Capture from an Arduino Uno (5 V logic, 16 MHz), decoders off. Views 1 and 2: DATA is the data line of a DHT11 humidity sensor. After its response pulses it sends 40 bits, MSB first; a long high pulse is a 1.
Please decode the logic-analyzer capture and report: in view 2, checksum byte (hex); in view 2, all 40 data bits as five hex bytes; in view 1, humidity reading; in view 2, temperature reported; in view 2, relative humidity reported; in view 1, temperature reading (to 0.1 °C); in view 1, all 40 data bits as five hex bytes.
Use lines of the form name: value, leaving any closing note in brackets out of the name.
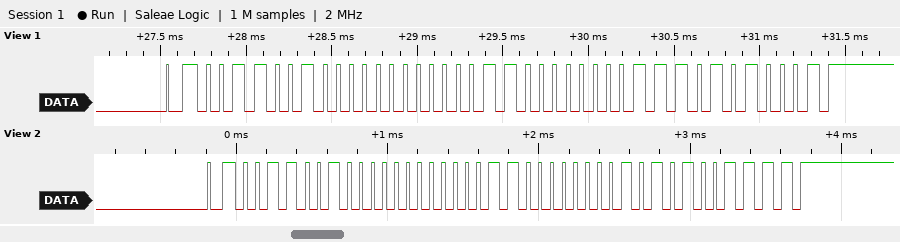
in view 2, checksum byte: 0x4F
in view 2, all 40 data bits as five hex bytes: 32 00 18 05 4F
in view 1, humidity reading: 50 %
in view 2, temperature reported: 24.5 °C
in view 2, relative humidity reported: 50 %
in view 1, temperature reading: 24.7 °C
in view 1, all 40 data bits as five hex bytes: 32 00 18 07 51
